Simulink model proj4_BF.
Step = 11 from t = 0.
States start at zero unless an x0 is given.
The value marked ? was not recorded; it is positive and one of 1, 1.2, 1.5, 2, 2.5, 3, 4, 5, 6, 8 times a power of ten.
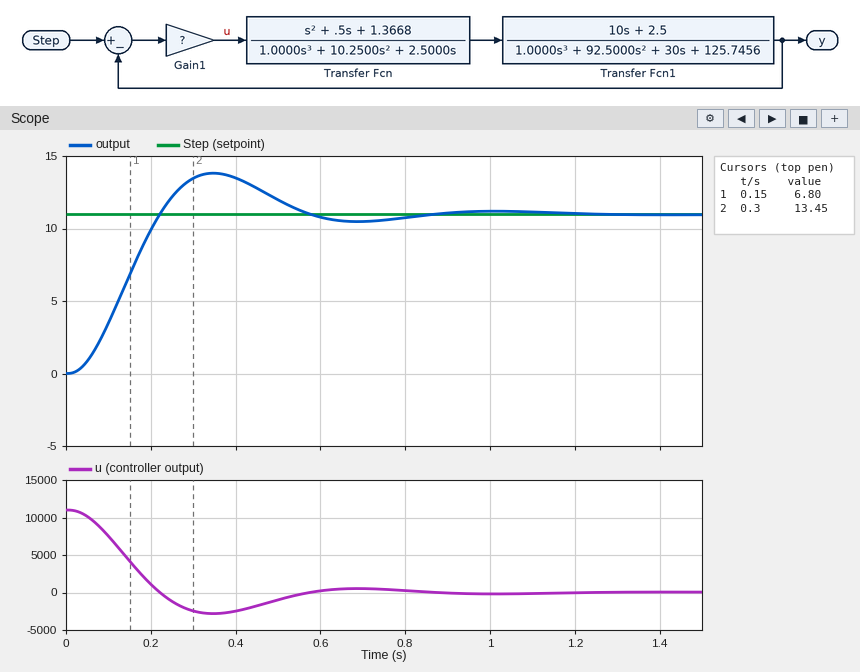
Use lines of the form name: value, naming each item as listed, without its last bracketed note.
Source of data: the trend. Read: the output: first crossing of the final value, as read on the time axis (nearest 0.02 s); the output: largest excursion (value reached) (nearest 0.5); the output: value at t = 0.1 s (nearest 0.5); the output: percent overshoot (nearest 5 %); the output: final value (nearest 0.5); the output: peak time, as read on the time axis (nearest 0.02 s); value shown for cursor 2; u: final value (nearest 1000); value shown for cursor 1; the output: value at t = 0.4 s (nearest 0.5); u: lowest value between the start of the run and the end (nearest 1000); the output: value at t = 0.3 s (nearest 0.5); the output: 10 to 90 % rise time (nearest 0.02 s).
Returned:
the output: first crossing of the final value, as read on the time axis: 0.22 s
the output: largest excursion (value reached): 14.0
the output: value at t = 0.1 s: 3.5
the output: percent overshoot: 25 %
the output: final value: 11.0
the output: peak time, as read on the time axis: 0.34 s
value shown for cursor 2: 13.45
u: final value: 0
value shown for cursor 1: 6.80
the output: value at t = 0.4 s: 13.5
u: lowest value between the start of the run and the end: -3000
the output: value at t = 0.3 s: 13.5
the output: 10 to 90 % rise time: 0.14 s
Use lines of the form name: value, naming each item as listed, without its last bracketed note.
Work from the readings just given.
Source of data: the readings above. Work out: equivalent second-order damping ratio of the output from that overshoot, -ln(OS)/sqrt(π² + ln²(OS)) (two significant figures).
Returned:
equivalent second-order damping ratio of the output from that overshoot, -ln(OS)/sqrt(π² + ln²(OS)): 0.40
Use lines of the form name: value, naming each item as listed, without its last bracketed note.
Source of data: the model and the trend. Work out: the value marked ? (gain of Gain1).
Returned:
the value marked ?: 1000
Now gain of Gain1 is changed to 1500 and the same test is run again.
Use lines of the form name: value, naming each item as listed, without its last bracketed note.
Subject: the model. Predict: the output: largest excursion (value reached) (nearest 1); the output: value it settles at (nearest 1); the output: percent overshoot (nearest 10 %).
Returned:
the output: largest excursion (value reached): 15
the output: value it settles at: 11
the output: percent overshoot: 40 %
